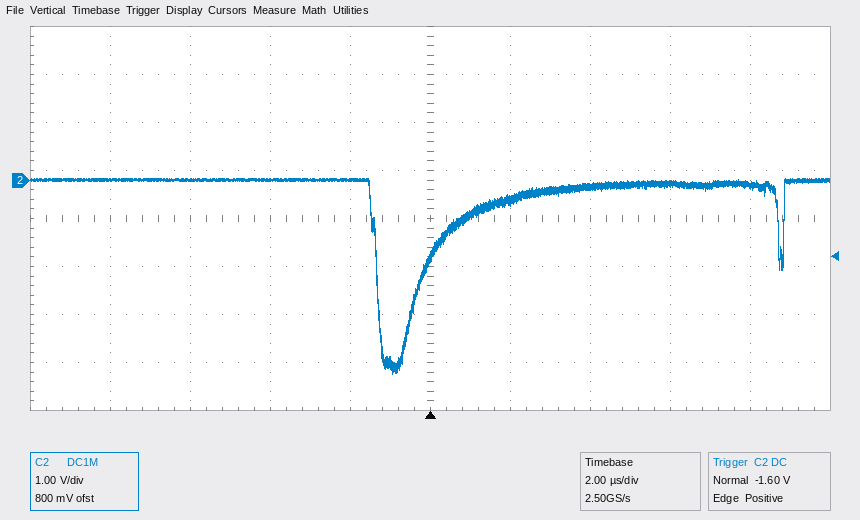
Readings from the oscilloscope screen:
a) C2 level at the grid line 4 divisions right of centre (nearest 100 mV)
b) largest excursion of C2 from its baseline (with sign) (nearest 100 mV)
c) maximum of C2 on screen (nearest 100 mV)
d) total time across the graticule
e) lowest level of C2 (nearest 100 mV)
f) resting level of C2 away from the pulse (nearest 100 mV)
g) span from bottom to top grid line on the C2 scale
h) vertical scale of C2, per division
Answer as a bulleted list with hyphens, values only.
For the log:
- -100 mV
- -4.0 V
- 0.0 V
- 20 µs
- -4.0 V
- 0.0 V
- 8 V
- 1 V
